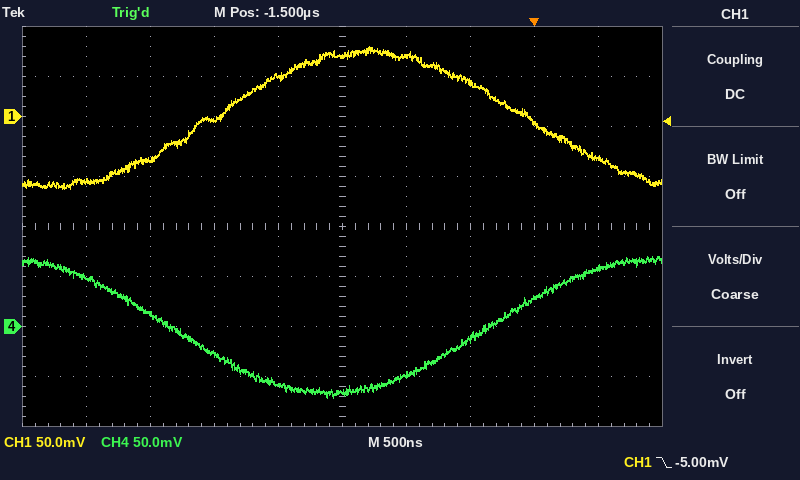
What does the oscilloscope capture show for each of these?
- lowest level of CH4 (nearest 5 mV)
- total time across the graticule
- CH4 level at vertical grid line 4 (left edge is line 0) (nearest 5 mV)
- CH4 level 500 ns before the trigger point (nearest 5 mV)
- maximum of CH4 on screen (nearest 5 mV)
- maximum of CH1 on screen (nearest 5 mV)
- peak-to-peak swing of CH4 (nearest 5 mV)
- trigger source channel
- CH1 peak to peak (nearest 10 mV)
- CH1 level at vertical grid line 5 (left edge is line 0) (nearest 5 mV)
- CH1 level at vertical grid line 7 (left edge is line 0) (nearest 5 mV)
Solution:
-70 mV
5 µs
-60 mV
-10 mV
70 mV
70 mV
140 mV
CH1
140 mV
60 mV
35 mV
